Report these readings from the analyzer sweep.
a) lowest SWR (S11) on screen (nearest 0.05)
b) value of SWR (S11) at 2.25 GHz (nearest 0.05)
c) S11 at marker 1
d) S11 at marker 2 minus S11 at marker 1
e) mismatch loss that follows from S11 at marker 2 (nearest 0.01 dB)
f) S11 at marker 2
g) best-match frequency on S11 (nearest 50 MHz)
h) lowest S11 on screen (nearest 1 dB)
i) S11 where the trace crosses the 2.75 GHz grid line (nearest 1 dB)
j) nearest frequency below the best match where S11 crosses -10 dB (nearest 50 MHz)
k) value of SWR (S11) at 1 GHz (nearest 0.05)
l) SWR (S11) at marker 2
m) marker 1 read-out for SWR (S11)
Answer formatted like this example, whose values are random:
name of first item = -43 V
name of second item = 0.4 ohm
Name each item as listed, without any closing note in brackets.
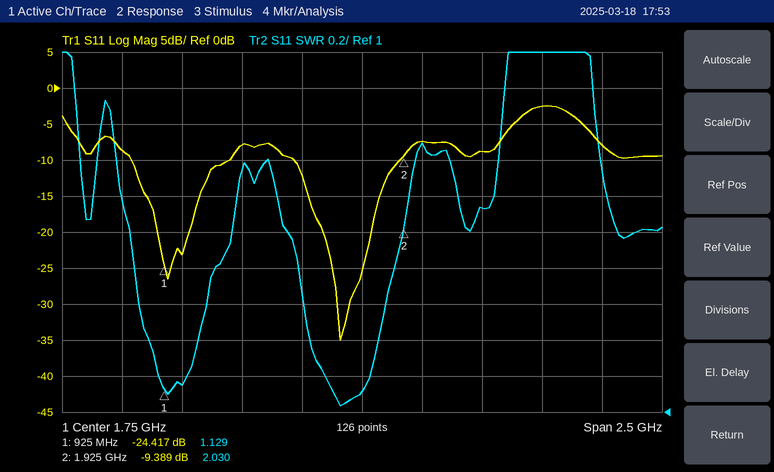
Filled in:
lowest SWR (S11) on screen = 1.05
value of SWR (S11) at 2.25 GHz = 2.15
S11 at marker 1 = -24.417 dB
S11 at marker 2 minus S11 at marker 1 = 15.028 dB
mismatch loss that follows from S11 at marker 2 = 0.53 dB
S11 at marker 2 = -9.389 dB
best-match frequency on S11 = 1.65 GHz
lowest S11 on screen = -35 dB
S11 where the trace crosses the 2.75 GHz grid line = -8 dB
nearest frequency below the best match where S11 crosses -10 dB = 1.45 GHz
value of SWR (S11) at 1 GHz = 1.15
SWR (S11) at marker 2 = 2.030
marker 1 read-out for SWR = 1.129
